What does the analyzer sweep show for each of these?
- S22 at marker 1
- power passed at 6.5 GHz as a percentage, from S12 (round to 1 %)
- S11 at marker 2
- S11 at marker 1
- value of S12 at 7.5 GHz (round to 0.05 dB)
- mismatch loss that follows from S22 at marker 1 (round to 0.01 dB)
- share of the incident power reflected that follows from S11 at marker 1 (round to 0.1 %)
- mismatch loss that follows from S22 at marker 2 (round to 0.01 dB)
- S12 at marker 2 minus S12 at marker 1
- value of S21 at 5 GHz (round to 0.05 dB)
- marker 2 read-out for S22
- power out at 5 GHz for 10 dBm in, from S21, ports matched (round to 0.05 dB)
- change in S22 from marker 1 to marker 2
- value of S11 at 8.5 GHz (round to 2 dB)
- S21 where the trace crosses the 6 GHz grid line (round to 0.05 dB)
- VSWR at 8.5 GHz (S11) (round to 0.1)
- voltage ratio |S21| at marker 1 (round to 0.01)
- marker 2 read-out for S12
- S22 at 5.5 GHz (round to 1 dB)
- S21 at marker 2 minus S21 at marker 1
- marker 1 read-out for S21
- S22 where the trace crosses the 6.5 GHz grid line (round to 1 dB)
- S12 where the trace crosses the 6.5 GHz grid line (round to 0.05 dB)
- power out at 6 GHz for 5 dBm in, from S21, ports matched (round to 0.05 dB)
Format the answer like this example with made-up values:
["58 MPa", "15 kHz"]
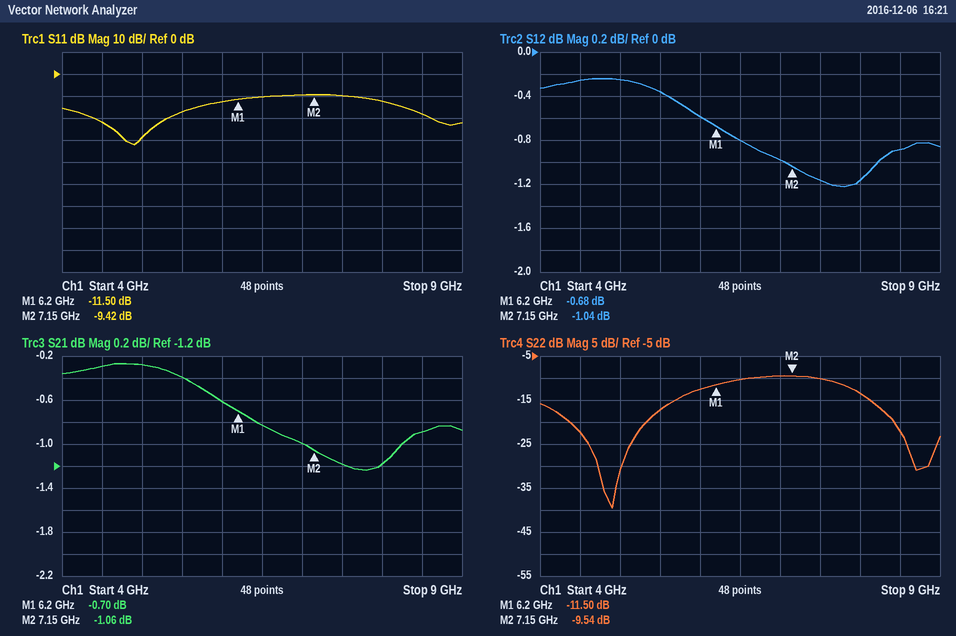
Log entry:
["-11.50 dB", "83 %", "-9.42 dB", "-11.50 dB", "-1.15 dB", "0.32 dB", "7.1 %", "0.51 dB", "-0.36 dB", "-0.30 dB", "-9.54 dB", "9.70 dBm", "1.96 dB", "-18 dB", "-0.60 dB", "1.3", "0.92", "-1.04 dB", "-17 dB", "-0.36 dB", "-0.70 dB", "-10 dB", "-0.80 dB", "4.40 dBm"]
